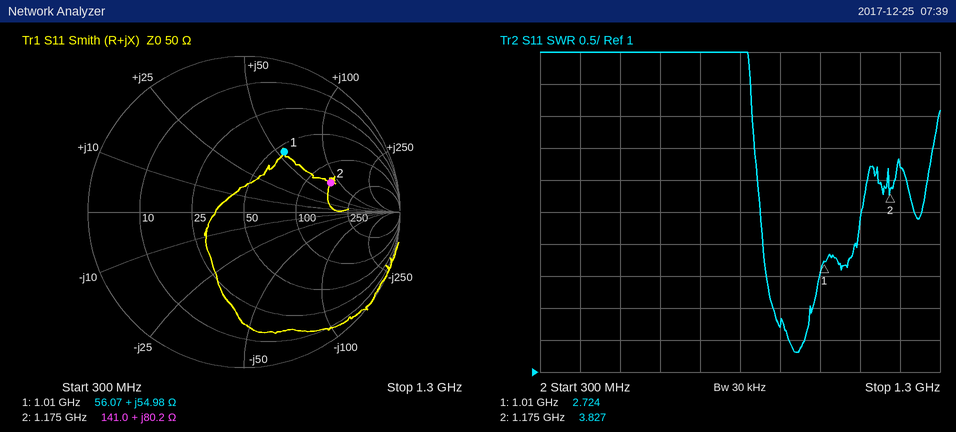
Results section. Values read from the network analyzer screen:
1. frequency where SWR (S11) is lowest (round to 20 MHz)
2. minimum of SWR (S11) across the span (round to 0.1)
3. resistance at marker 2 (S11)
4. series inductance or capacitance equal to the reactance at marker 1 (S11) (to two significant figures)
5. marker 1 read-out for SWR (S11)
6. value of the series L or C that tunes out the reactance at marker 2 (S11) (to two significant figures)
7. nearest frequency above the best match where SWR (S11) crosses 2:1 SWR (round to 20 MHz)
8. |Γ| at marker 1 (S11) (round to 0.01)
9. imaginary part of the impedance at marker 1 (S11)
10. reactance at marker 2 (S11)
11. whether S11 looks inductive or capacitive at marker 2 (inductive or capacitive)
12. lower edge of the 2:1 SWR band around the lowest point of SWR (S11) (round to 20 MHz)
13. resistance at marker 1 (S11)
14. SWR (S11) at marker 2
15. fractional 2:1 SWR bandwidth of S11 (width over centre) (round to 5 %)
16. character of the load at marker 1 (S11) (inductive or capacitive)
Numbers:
940 MHz
1.3
141.0 Ω
8.7 nH
2.724
1.7 pF
980 MHz
0.46
+54.98 Ω
+80.2 Ω
inductive
880 MHz
56.07 Ω
3.827
10 %
inductive
